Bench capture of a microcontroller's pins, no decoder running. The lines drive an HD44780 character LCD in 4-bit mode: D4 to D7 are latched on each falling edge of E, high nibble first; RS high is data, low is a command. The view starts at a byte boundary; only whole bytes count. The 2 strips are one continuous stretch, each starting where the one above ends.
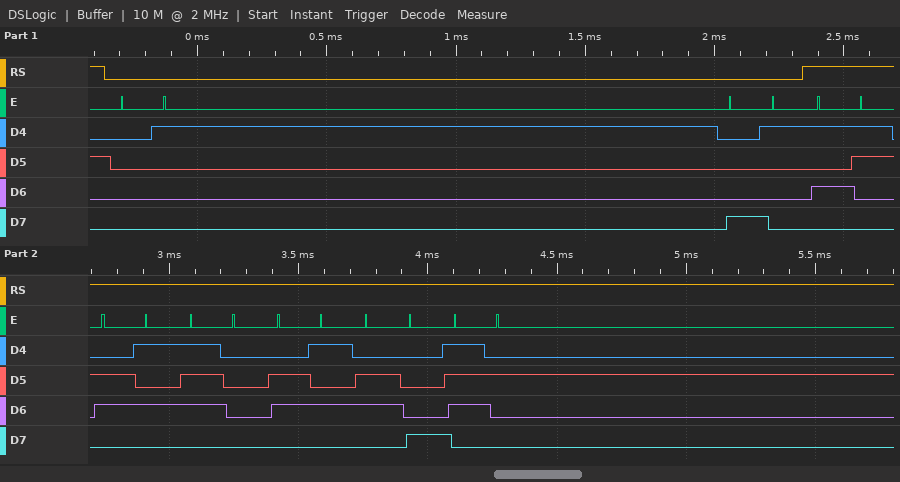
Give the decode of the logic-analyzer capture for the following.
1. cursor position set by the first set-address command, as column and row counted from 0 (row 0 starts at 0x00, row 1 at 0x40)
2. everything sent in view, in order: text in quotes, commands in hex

column 1, row 0
0x01 0x81 "Sepehr"
